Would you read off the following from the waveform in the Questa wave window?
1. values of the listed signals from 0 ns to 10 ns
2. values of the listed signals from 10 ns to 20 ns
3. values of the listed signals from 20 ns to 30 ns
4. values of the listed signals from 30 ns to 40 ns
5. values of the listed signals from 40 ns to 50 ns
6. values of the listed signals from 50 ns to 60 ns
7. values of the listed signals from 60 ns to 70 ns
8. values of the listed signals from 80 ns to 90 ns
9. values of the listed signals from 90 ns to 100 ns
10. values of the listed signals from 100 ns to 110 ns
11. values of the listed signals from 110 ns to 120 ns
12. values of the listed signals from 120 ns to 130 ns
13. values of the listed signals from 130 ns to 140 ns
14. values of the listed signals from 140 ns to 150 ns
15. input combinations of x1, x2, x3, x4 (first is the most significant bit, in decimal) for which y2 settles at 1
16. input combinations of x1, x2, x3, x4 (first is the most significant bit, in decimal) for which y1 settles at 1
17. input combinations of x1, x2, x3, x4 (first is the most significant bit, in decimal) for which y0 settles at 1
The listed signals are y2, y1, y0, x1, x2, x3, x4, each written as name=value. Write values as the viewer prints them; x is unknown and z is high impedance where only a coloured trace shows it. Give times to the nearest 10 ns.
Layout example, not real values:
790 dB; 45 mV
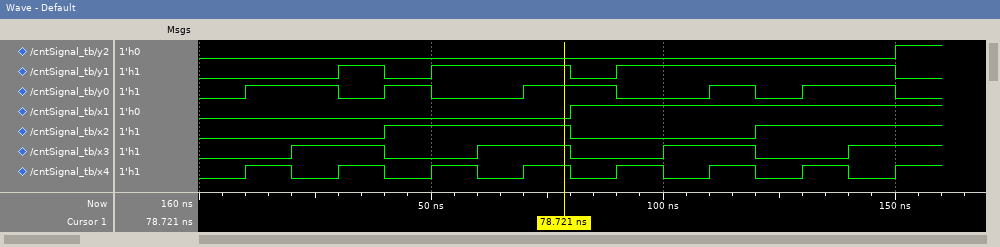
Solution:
y2=0, y1=0, y0=0, x1=0, x2=0, x3=0, x4=0; y2=0, y1=0, y0=1, x1=0, x2=0, x3=0, x4=1; y2=0, y1=0, y0=1, x1=0, x2=0, x3=1, x4=0; y2=0, y1=1, y0=0, x1=0, x2=0, x3=1, x4=1; y2=0, y1=0, y0=1, x1=0, x2=1, x3=0, x4=0; y2=0, y1=1, y0=0, x1=0, x2=1, x3=0, x4=1; y2=0, y1=1, y0=0, x1=0, x2=1, x3=1, x4=0; y2=0, y1=0, y0=1, x1=1, x2=0, x3=0, x4=0; y2=0, y1=1, y0=0, x1=1, x2=0, x3=0, x4=1; y2=0, y1=1, y0=0, x1=1, x2=0, x3=1, x4=0; y2=0, y1=1, y0=1, x1=1, x2=0, x3=1, x4=1; y2=0, y1=1, y0=0, x1=1, x2=1, x3=0, x4=0; y2=0, y1=1, y0=1, x1=1, x2=1, x3=0, x4=1; y2=0, y1=1, y0=1, x1=1, x2=1, x3=1, x4=0; 15; 3, 5, 6, 7, 9, 10, 11, 12, 13, 14; 1, 2, 4, 7, 8, 11, 13, 14
